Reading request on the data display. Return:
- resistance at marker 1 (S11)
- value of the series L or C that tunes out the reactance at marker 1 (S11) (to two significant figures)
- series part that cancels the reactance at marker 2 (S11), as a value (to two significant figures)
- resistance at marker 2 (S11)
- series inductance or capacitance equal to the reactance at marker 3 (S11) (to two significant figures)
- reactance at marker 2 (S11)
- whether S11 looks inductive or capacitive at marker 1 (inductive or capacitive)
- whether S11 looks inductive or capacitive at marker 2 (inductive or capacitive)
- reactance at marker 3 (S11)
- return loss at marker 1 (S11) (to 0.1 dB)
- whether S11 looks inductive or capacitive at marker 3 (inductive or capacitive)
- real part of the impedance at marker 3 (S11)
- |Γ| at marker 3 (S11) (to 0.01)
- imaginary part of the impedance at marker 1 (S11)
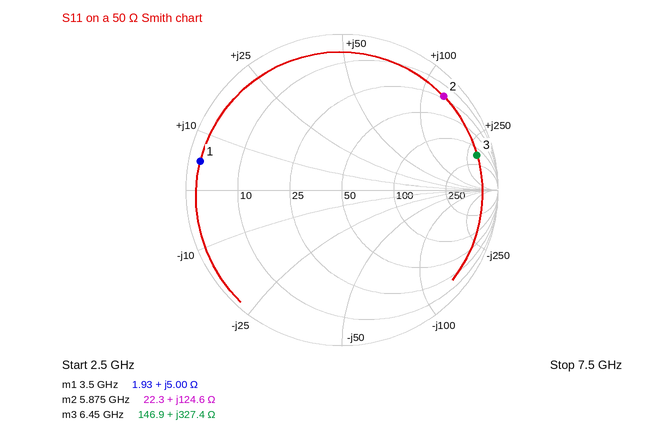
1.93 Ω
9.1 pF
220 fF
22.3 Ω
8.1 nH
+124.6 Ω
inductive
inductive
+327.4 Ω
0.7 dB
inductive
146.9 Ω
0.89
+5.00 Ω
